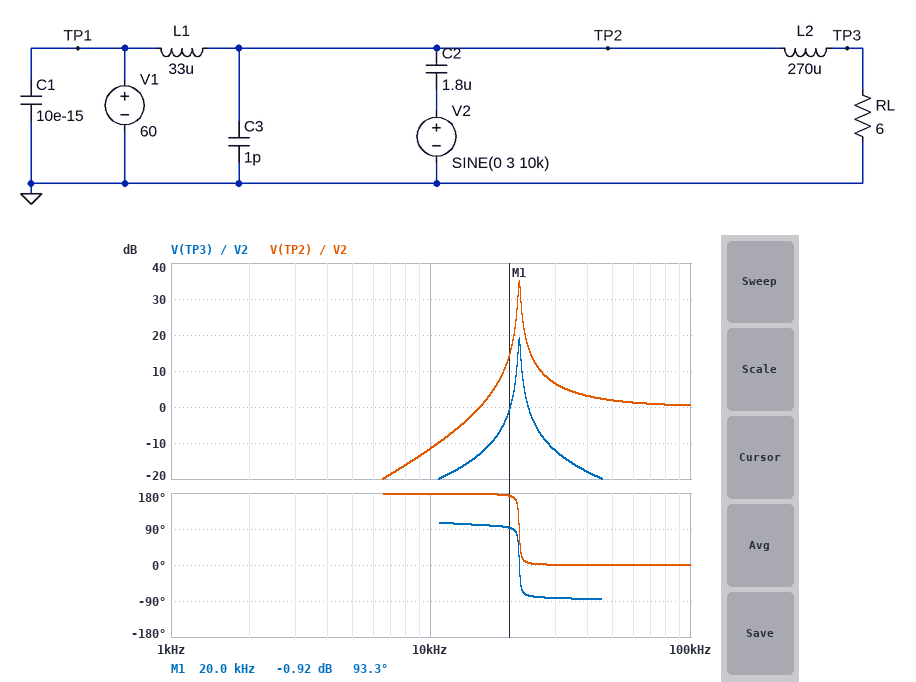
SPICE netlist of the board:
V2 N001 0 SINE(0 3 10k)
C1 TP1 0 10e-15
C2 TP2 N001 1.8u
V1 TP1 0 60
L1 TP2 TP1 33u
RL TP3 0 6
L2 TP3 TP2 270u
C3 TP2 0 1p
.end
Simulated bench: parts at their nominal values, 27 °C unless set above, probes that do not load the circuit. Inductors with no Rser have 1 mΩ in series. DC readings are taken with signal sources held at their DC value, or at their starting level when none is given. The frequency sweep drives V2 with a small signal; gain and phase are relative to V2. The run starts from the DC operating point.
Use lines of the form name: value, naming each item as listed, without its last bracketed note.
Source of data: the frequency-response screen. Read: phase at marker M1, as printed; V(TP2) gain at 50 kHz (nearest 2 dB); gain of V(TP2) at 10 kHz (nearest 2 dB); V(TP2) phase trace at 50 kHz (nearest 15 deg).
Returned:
phase at marker M1, as printed: 93.3 deg
V(TP2) gain at 50 kHz: 2 dB
gain of V(TP2) at 10 kHz: -12 dB
V(TP2) phase trace at 50 kHz: 0 deg
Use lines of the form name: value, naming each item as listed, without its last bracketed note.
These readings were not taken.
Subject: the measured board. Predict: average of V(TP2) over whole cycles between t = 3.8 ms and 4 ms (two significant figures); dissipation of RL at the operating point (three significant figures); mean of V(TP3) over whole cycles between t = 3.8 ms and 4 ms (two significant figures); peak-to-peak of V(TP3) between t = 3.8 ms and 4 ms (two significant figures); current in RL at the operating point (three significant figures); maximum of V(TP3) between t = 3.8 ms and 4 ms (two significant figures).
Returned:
average of V(TP2) over whole cycles between t = 3.8 ms and 4 ms: 60 V
dissipation of RL at the operating point: 600 W
mean of V(TP3) over whole cycles between t = 3.8 ms and 4 ms: 60 V
peak-to-peak of V(TP3) between t = 3.8 ms and 4 ms: 540 mV
current in RL at the operating point: 10.0 A
maximum of V(TP3) between t = 3.8 ms and 4 ms: 60 V
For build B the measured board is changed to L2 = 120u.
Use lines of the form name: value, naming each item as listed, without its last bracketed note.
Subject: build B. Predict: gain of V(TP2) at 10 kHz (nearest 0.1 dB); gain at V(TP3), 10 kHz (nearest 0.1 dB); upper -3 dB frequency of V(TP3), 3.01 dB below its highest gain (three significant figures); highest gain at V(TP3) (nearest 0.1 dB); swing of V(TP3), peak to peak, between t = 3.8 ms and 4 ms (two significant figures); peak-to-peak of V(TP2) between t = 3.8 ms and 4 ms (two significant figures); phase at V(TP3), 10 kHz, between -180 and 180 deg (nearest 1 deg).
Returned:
gain of V(TP2) at 10 kHz: -12.1 dB
gain at V(TP3), 10 kHz: -16.2 dB
upper -3 dB frequency of V(TP3), 3.01 dB below its highest gain: 23.9 kHz
highest gain at V(TP3): 13.6 dB
swing of V(TP3), peak to peak, between t = 3.8 ms and 4 ms: 930 mV
peak-to-peak of V(TP2) between t = 3.8 ms and 4 ms: 1.5 V
phase at V(TP3), 10 kHz, between -180 and 180 deg: 120 deg
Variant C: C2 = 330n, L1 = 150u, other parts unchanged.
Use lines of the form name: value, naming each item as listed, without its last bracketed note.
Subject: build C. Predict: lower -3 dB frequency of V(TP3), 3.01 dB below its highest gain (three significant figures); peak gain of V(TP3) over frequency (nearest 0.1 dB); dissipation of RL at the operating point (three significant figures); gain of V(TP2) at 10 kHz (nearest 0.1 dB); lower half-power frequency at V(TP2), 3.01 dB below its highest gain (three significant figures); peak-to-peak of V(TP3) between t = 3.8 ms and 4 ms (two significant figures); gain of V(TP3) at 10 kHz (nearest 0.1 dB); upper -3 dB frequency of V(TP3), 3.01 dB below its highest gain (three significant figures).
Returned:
lower -3 dB frequency of V(TP3), 3.01 dB below its highest gain: 27.5 kHz
peak gain of V(TP3) over frequency: 9.0 dB
dissipation of RL at the operating point: 600 W
gain of V(TP2) at 10 kHz: -16.5 dB
lower half-power frequency at V(TP2), 3.01 dB below its highest gain: 27.6 kHz
peak-to-peak of V(TP3) between t = 3.8 ms and 4 ms: 300 mV
gain of V(TP3) at 10 kHz: -26.1 dB
upper -3 dB frequency of V(TP3), 3.01 dB below its highest gain: 28.8 kHz
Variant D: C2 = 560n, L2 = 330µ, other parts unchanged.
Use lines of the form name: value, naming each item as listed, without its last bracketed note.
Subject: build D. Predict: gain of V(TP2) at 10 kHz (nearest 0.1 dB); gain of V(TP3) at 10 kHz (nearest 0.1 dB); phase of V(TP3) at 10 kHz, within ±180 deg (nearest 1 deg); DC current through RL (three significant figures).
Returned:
gain of V(TP2) at 10 kHz: -22.9 dB
gain of V(TP3) at 10 kHz: -34.0 dB
phase of V(TP3) at 10 kHz, within ±180 deg: 105 deg
DC current through RL: 10.0 A
